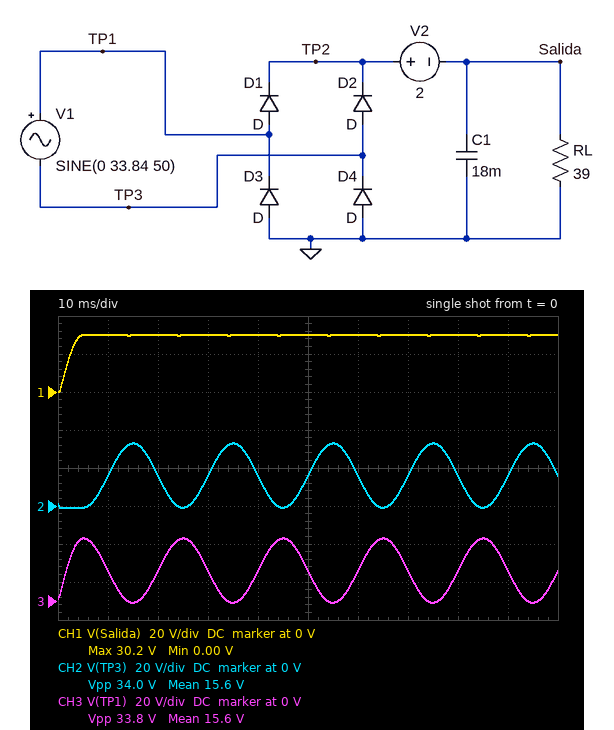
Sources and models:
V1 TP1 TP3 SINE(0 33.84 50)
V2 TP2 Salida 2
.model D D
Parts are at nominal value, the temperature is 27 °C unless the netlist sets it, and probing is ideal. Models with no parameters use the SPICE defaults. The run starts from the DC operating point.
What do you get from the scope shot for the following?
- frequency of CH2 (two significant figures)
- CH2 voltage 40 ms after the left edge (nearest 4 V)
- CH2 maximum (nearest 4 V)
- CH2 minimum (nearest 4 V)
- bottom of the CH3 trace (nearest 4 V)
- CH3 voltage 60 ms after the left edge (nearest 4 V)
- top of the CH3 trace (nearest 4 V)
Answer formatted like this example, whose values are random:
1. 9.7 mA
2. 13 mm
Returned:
1. 50 Hz
2. 16 V
3. 32 V
4. 0 V
5. 0 V
6. 16 V
7. 32 V
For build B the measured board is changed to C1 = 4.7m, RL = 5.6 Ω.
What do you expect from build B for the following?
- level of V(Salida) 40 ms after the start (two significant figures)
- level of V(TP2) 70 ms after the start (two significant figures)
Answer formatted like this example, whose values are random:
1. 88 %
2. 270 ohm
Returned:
1. 25 V
2. 27 V
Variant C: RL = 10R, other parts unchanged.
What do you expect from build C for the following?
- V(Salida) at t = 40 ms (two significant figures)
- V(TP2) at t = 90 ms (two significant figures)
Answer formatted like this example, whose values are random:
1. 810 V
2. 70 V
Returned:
1. 29 V
2. 31 V
